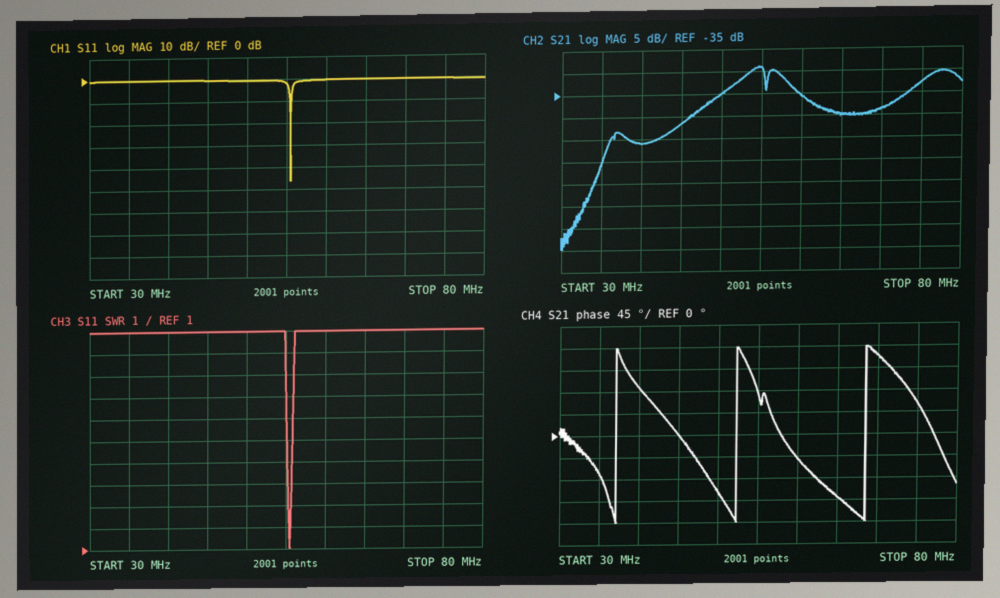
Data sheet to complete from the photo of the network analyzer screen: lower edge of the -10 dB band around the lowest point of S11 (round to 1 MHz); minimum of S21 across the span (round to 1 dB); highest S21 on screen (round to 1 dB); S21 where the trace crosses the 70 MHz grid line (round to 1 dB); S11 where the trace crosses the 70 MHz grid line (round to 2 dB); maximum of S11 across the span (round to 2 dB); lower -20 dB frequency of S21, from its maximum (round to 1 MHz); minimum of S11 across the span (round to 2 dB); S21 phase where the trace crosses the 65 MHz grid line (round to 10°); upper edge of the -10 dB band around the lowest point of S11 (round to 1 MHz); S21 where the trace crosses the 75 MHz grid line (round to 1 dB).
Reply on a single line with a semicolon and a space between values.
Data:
55 MHz; -70 dB; -29 dB; -39 dB; 0 dB; 0 dB; 35 MHz; -46 dB; -130°; 56 MHz; -33 dB
